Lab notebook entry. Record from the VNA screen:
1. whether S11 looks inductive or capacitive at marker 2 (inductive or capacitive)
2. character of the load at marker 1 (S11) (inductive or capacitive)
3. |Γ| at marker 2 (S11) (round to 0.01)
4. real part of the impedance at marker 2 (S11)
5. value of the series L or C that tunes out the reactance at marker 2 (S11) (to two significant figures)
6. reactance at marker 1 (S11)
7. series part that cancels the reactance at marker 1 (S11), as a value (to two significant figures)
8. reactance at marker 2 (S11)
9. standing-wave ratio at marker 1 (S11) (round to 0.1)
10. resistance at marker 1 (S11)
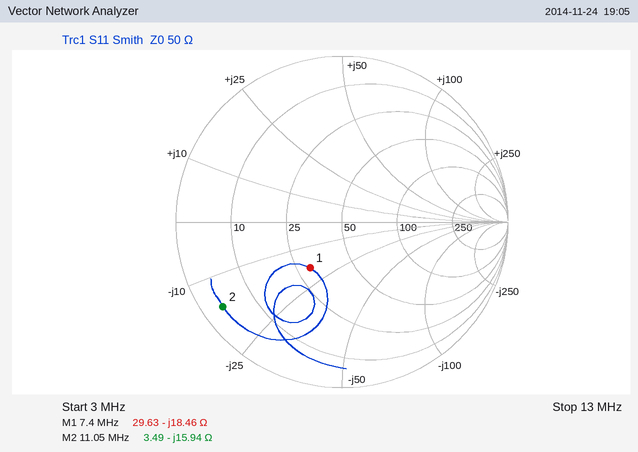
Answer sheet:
capacitive
capacitive
0.88
3.49 Ω
230 nH
-18.46 Ω
400 nH
-15.94 Ω
2.0
29.63 Ω
